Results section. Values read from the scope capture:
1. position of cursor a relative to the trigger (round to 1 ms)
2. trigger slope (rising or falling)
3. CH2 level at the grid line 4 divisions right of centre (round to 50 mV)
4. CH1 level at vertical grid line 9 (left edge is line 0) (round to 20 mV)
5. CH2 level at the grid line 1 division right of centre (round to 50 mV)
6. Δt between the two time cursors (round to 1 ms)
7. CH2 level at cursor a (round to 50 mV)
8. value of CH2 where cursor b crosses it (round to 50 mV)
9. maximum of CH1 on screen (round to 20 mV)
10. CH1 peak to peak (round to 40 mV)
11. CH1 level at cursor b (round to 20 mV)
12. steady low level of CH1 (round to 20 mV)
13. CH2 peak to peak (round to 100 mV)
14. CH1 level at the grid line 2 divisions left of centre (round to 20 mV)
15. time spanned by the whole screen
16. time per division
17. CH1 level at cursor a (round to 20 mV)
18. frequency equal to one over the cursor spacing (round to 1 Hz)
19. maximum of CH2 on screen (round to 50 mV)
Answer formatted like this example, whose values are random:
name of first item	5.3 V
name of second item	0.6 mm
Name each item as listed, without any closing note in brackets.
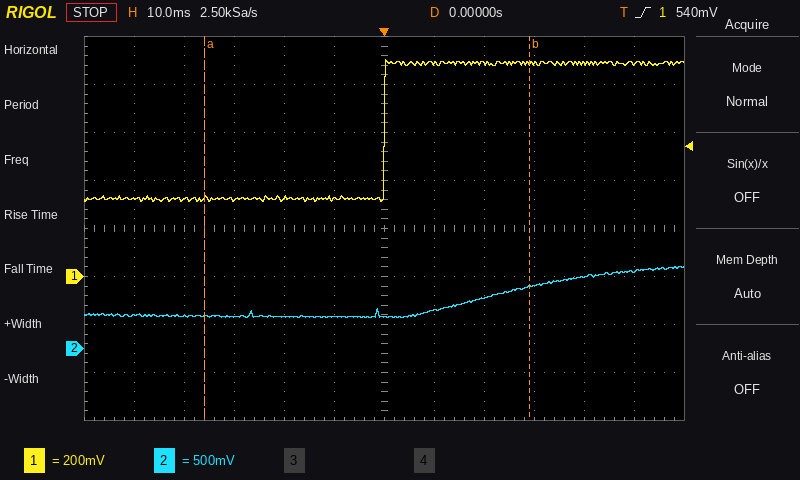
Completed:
position of cursor a relative to the trigger	-36 ms
trigger slope	rising
CH2 level at the grid line 4 divisions right of centre	750 mV
CH1 level at vertical grid line 9 (left edge is line 0)	880 mV
CH2 level at the grid line 1 division right of centre	400 mV
Δt between the two time cursors	65 ms
CH2 level at cursor a	350 mV
value of CH2 where cursor b crosses it	650 mV
maximum of CH1 on screen	900 mV
CH1 peak to peak	600 mV
CH1 level at cursor b	880 mV
steady low level of CH1	320 mV
CH2 peak to peak	500 mV
CH1 level at the grid line 2 divisions left of centre	320 mV
time spanned by the whole screen	120 ms
time per division	10 ms
CH1 level at cursor a	320 mV
frequency equal to one over the cursor spacing	15 Hz
maximum of CH2 on screen	850 mV
